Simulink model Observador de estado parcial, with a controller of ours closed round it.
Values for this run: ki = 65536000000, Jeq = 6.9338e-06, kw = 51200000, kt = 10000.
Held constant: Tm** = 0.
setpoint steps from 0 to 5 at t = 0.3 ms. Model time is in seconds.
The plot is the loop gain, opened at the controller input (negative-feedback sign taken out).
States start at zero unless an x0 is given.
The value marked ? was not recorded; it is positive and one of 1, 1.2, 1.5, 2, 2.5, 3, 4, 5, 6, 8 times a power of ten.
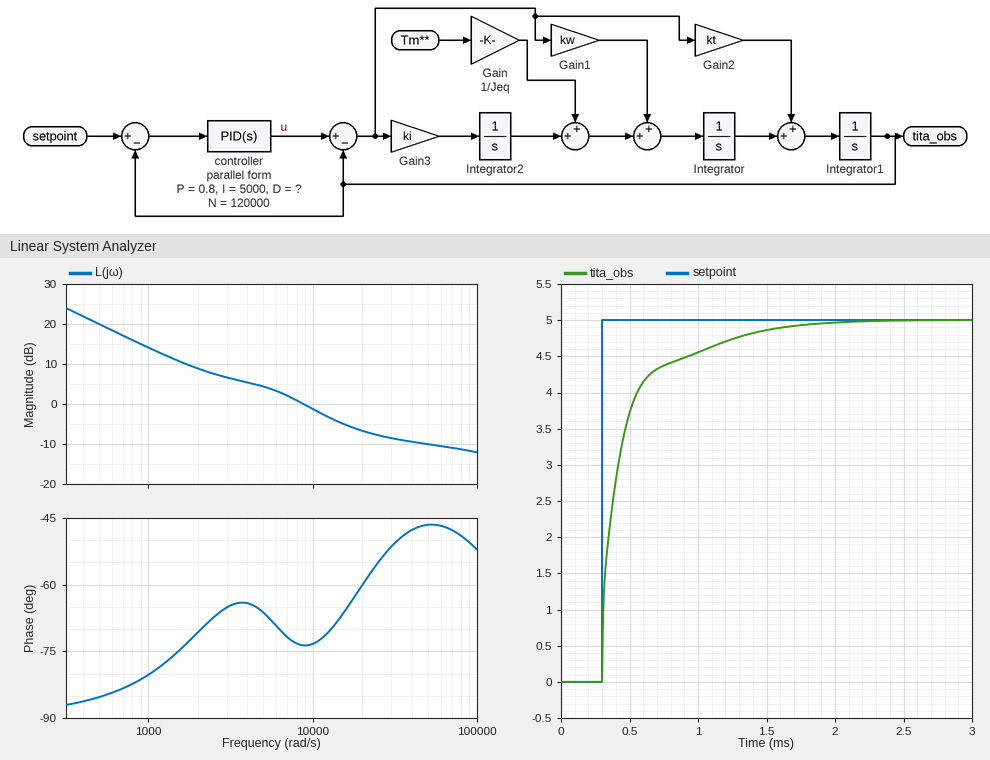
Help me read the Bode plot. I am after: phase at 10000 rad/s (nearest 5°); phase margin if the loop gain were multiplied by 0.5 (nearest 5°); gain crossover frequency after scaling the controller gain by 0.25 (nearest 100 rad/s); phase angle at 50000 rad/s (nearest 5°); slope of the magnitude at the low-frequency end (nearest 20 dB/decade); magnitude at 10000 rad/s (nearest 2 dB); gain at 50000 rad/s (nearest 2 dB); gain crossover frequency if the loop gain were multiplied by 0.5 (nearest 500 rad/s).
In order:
-75°
115°
1300 rad/s
-45°
-20 dB/decade
-2 dB
-10 dB
3500 rad/s
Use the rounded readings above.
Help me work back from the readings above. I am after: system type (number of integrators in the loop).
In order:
1
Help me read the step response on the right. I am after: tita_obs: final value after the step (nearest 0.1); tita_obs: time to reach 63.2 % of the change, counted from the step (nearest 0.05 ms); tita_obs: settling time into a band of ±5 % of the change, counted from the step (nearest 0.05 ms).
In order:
5.0
0.15 ms
0.95 ms
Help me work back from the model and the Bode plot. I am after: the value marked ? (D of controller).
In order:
2.5e-05
